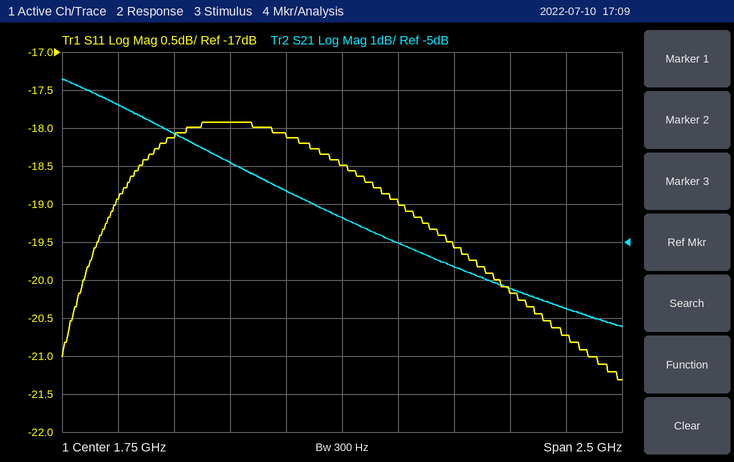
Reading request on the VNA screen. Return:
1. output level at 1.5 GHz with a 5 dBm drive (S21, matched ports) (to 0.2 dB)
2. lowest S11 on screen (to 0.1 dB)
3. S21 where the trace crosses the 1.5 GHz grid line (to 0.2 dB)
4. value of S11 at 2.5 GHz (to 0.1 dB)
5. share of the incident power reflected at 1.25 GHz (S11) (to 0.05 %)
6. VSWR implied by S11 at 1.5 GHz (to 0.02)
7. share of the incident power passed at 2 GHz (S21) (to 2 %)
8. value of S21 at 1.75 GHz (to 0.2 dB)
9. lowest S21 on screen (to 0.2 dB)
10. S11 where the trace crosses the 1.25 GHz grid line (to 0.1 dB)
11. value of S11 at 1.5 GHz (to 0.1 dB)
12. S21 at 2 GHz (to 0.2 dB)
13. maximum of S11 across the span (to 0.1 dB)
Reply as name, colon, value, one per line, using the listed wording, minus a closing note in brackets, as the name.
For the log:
output level at 1.5 GHz with a 5 dBm drive (S21, matched ports): 1.4 dBm
lowest S11 on screen: -21.3 dB
S21 where the trace crosses the 1.5 GHz grid line: -3.6 dB
value of S11 at 2.5 GHz: -20.2 dB
share of the incident power reflected at 1.25 GHz (S11): 1.60 %
VSWR implied by S11 at 1.5 GHz: 1.28
share of the incident power passed at 2 GHz (S21): 32 %
value of S21 at 1.75 GHz: -4.4 dB
lowest S21 on screen: -7.2 dB
S11 where the trace crosses the 1.25 GHz grid line: -17.9 dB
value of S11 at 1.5 GHz: -18.1 dB
S21 at 2 GHz: -5.0 dB
maximum of S11 across the span: -17.9 dB
